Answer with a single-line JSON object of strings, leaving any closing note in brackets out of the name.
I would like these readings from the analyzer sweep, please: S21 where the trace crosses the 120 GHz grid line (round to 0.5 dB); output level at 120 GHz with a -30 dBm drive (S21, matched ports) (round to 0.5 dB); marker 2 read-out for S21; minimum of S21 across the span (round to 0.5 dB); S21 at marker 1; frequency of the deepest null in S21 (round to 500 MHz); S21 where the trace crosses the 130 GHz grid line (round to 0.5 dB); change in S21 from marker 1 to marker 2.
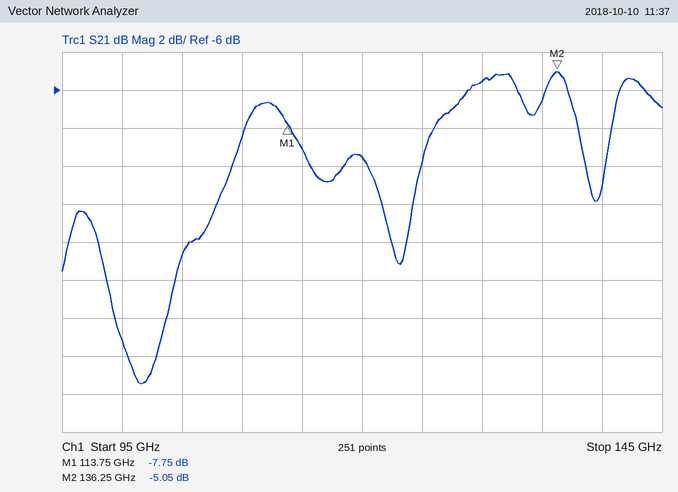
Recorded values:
{"S21 where the trace crosses the 120 GHz grid line": "-9.5 dB", "output level at 120 GHz with a -30 dBm drive (S21, matched ports)": "-39.5 dBm", "marker 2 read-out for S21": "-5.05 dB", "minimum of S21 across the span": "-21.5 dB", "S21 at marker 1": "-7.75 dB", "frequency of the deepest null in S21": "101.5 GHz", "S21 where the trace crosses the 130 GHz grid line": "-5.5 dB", "change in S21 from marker 1 to marker 2": "2.70 dB"}
